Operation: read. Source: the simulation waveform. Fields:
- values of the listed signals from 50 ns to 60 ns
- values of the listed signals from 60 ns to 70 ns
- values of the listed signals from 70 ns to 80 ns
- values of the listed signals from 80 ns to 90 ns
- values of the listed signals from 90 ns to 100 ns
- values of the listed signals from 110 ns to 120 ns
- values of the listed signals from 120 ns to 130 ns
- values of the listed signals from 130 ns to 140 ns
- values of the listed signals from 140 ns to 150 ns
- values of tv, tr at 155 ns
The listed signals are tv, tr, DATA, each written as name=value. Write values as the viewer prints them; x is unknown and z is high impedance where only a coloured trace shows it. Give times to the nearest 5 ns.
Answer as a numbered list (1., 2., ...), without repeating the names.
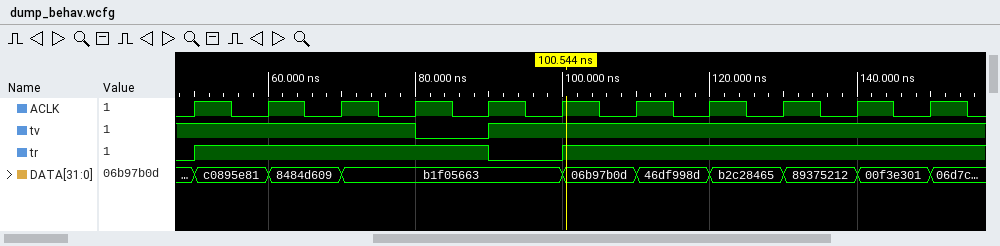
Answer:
1. tv=1, tr=1, DATA=c0895e81
2. tv=1, tr=1, DATA=8484d609
3. tv=1, tr=1, DATA=b1f05663
4. tv=0, tr=1, DATA=b1f05663
5. tv=1, tr=0, DATA=b1f05663
6. tv=1, tr=1, DATA=46df998d
7. tv=1, tr=1, DATA=b2c28465
8. tv=1, tr=1, DATA=89375212
9. tv=1, tr=1, DATA=00f3e301
10. tv=1, tr=1
